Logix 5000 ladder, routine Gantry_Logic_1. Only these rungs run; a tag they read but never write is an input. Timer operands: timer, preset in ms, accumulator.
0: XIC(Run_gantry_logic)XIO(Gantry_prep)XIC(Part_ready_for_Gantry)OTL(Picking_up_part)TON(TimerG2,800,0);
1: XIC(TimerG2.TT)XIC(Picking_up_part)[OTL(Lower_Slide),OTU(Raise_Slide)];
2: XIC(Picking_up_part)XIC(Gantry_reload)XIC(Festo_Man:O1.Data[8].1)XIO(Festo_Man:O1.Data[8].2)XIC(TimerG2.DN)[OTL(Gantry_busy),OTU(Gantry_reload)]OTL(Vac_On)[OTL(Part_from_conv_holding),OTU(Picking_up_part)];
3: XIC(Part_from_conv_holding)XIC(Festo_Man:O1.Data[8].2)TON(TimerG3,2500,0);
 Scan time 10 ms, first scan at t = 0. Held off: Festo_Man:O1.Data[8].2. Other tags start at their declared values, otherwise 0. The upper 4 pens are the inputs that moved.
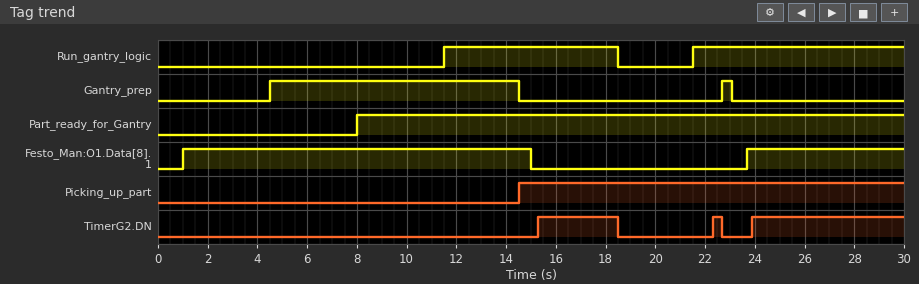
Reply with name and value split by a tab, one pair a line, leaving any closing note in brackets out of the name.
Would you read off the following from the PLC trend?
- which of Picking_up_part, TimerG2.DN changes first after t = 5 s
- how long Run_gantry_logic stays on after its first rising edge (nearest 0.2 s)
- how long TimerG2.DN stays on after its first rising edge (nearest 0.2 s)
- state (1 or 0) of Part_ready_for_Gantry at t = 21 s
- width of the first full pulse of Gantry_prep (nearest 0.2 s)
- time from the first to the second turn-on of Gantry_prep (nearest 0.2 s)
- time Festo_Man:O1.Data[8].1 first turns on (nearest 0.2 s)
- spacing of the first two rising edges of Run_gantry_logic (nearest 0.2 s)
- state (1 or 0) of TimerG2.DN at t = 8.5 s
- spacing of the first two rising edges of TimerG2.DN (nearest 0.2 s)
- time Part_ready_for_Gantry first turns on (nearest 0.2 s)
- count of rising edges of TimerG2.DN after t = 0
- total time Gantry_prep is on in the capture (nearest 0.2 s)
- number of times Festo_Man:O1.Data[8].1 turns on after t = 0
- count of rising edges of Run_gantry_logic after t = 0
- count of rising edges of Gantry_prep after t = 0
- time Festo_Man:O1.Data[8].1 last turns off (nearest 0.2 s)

which of Picking_up_part, TimerG2.DN changes first after t = 5 s	Picking_up_part
how long Run_gantry_logic stays on after its first rising edge	7.0 s
how long TimerG2.DN stays on after its first rising edge	3.2 s
state (1 or 0) of Part_ready_for_Gantry at t = 21 s	1
width of the first full pulse of Gantry_prep	10.0 s
time from the first to the second turn-on of Gantry_prep	18.2 s
time Festo_Man:O1.Data[8].1 first turns on	1.0 s
spacing of the first two rising edges of Run_gantry_logic	10.0 s
state (1 or 0) of TimerG2.DN at t = 8.5 s	0
spacing of the first two rising edges of TimerG2.DN	7.0 s
time Part_ready_for_Gantry first turns on	8.0 s
count of rising edges of TimerG2.DN after t = 0	3
total time Gantry_prep is on in the capture	10.4 s
number of times Festo_Man:O1.Data[8].1 turns on after t = 0	2
count of rising edges of Run_gantry_logic after t = 0	2
count of rising edges of Gantry_prep after t = 0	2
time Festo_Man:O1.Data[8].1 last turns off	15.0 s
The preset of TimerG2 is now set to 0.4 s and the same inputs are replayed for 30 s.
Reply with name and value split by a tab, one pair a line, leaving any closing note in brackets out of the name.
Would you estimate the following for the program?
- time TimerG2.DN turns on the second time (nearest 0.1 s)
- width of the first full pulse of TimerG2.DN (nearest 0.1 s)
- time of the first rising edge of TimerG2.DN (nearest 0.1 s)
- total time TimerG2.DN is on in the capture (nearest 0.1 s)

time TimerG2.DN turns on the second time	21.9 s
width of the first full pulse of TimerG2.DN	3.6 s
time of the first rising edge of TimerG2.DN	14.9 s
total time TimerG2.DN is on in the capture	10.9 s
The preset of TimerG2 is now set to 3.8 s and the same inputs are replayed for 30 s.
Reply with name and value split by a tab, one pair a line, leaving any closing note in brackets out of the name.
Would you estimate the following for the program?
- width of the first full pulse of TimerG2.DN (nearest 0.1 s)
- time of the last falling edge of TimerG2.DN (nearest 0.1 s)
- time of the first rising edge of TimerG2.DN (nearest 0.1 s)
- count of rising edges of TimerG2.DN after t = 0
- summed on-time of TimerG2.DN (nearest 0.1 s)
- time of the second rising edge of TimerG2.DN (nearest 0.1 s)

width of the first full pulse of TimerG2.DN	0.2 s
time of the last falling edge of TimerG2.DN	18.5 s
time of the first rising edge of TimerG2.DN	18.3 s
count of rising edges of TimerG2.DN after t = 0	2
summed on-time of TimerG2.DN	3.3 s
time of the second rising edge of TimerG2.DN	26.9 s
